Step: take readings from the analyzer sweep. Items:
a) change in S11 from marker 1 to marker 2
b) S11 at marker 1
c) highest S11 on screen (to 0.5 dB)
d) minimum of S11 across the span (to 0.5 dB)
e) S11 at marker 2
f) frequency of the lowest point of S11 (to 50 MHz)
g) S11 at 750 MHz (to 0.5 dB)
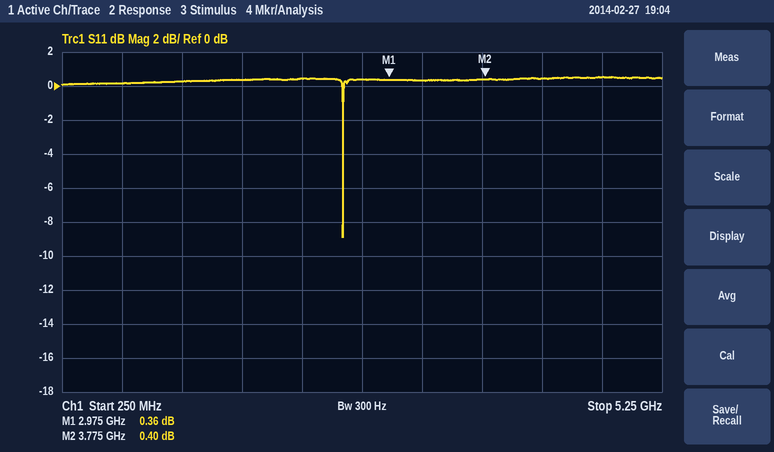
0.04 dB
0.36 dB
0.5 dB
-9.0 dB
0.40 dB
2.60 GHz
0.0 dB
